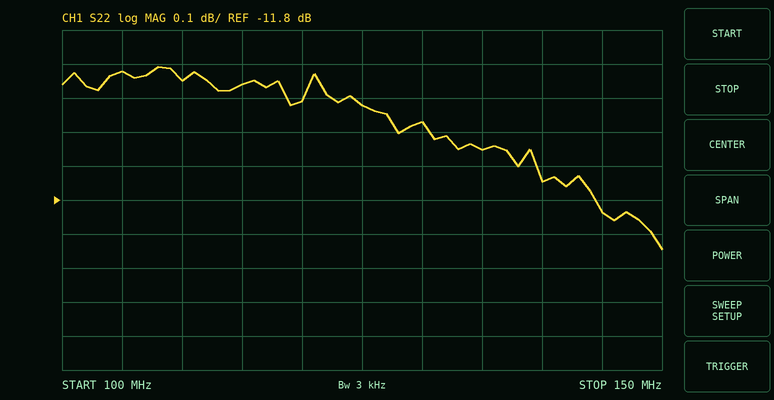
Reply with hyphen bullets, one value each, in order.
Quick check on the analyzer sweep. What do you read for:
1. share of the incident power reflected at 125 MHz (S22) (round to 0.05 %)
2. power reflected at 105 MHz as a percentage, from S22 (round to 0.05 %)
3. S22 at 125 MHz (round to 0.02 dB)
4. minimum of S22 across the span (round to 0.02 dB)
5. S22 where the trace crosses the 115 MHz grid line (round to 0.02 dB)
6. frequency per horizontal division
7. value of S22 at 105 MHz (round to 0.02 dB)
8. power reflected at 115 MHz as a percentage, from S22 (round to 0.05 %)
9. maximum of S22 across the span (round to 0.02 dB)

- 7.05 %
- 7.20 %
- -11.52 dB
- -11.94 dB
- -11.46 dB
- 5 MHz
- -11.42 dB
- 7.15 %
- -11.40 dB
